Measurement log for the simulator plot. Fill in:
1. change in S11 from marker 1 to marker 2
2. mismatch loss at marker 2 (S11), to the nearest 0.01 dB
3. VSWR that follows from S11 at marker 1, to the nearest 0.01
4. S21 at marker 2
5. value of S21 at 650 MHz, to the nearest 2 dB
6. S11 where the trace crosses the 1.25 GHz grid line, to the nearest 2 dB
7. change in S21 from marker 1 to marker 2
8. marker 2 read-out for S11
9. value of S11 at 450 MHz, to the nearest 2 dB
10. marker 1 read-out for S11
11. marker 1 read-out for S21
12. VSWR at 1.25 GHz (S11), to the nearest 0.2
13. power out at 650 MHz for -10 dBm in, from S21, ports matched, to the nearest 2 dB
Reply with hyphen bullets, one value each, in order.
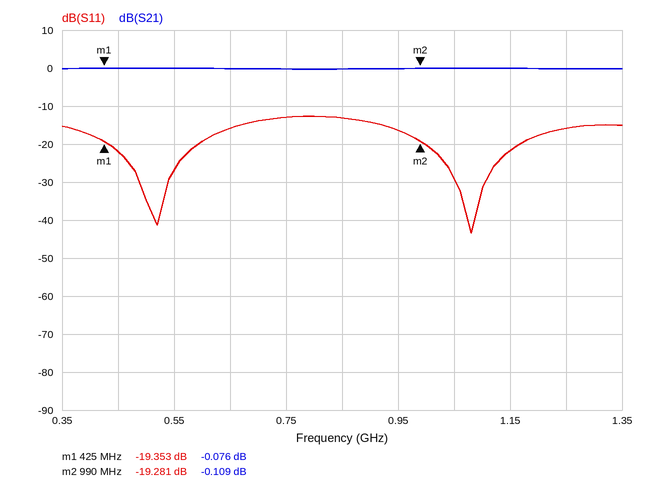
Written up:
- 0.072 dB
- 0.05 dB
- 1.24
- -0.109 dB
- 0 dB
- -16 dB
- -0.033 dB
- -19.281 dB
- -22 dB
- -19.353 dB
- -0.076 dB
- 1.4
- -10 dBm
